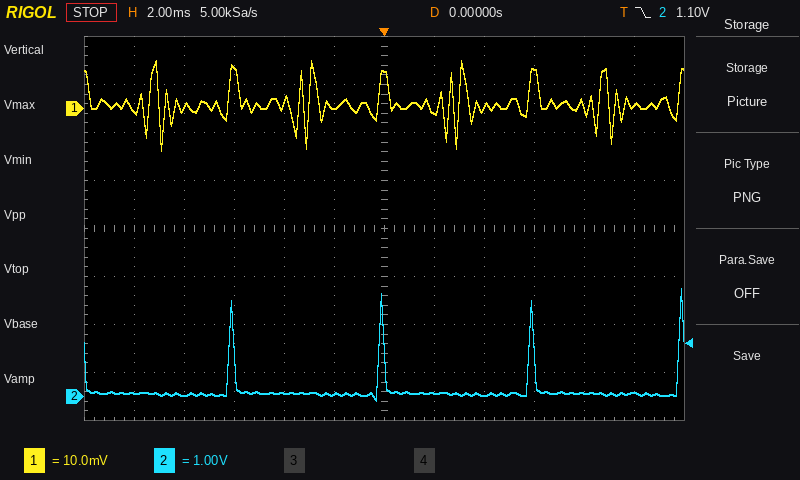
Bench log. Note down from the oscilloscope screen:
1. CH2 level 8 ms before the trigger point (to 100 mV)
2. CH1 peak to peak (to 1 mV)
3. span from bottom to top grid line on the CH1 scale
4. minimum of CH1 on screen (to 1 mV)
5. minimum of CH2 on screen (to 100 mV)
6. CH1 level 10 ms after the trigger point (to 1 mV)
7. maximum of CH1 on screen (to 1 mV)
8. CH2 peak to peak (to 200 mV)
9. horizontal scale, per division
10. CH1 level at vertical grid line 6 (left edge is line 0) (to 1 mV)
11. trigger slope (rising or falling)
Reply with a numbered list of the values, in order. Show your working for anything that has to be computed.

1. 0.0 V
2. 10 mV − (-9 mV) = 19 mV
3. 80 mV
4. -9 mV
5. -100 mV
6. 1 mV
7. 10 mV
8. 2.4 V
9. 2 ms
10. 7 mV
11. falling
